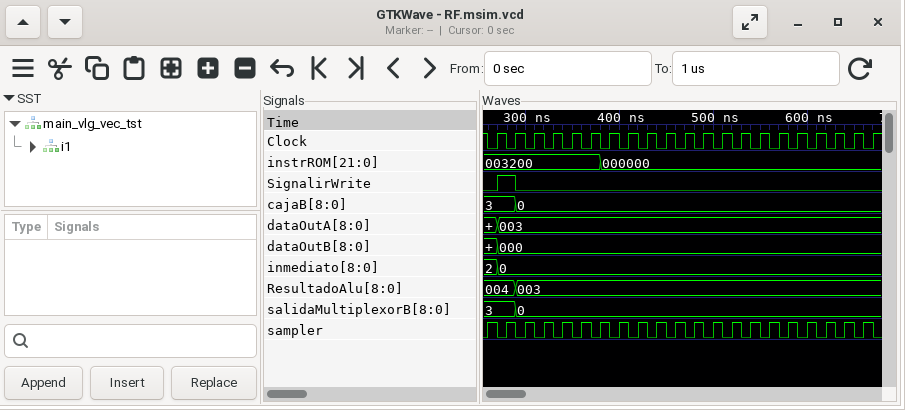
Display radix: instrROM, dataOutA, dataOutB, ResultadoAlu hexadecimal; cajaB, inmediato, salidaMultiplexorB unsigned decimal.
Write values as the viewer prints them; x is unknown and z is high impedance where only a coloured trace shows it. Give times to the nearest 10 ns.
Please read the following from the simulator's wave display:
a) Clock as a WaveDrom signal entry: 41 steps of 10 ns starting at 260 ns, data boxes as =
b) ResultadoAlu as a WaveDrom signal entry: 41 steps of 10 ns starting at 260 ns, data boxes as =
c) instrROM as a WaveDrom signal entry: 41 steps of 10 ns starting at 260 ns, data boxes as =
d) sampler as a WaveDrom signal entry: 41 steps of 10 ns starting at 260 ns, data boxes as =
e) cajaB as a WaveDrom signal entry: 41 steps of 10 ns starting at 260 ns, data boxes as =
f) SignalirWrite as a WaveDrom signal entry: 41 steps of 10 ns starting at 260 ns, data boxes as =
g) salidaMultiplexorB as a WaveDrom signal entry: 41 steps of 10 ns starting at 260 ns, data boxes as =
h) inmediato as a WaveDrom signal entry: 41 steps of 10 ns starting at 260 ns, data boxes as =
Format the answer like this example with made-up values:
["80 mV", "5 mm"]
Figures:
["{name: 'Clock', wave: '01010101010101010101010101010101010101010'}", "{name: 'ResultadoAlu', wave: '=..=.....................................', data: '004 003'}", "{name: 'instrROM', wave: '=...........=............................', data: '003200 000000'}", "{name: 'sampler', wave: '10101010101010101010101010101010101010101'}", "{name: 'cajaB', wave: '=..=.....................................', data: '3 0'}", "{name: 'SignalirWrite', wave: '01.0.....................................'}", "{name: 'salidaMultiplexorB', wave: '=..=.....................................', data: '3 0'}", "{name: 'inmediato', wave: '==.......................................', data: '2 0'}"]
